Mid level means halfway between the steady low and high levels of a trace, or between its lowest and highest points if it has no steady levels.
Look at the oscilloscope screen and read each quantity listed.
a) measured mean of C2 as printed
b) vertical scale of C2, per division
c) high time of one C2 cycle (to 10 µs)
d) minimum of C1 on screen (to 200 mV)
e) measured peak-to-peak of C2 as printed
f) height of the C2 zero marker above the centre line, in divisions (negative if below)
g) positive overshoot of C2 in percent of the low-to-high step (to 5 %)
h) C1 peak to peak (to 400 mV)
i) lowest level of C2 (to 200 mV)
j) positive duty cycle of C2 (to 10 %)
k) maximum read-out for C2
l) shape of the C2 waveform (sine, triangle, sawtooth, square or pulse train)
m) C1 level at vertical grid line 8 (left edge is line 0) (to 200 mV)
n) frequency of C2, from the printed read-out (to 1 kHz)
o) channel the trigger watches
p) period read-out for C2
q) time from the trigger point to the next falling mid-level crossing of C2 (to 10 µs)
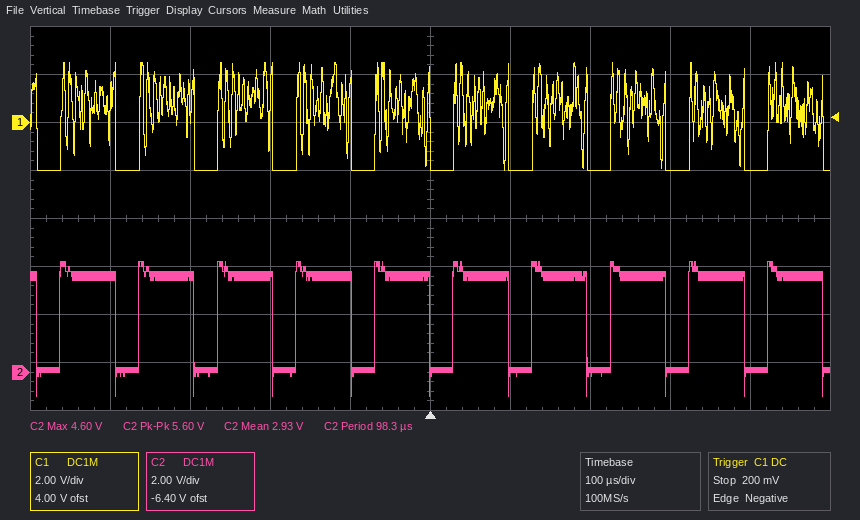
2.93 V
2 V
70 µs
-2.0 V
5.60 V
-3.2 div
15 %
4.4 V
-1.0 V
70 %
4.60 V
pulse train
-2.0 V
10 kHz
C1
98.3 µs
100 µs
